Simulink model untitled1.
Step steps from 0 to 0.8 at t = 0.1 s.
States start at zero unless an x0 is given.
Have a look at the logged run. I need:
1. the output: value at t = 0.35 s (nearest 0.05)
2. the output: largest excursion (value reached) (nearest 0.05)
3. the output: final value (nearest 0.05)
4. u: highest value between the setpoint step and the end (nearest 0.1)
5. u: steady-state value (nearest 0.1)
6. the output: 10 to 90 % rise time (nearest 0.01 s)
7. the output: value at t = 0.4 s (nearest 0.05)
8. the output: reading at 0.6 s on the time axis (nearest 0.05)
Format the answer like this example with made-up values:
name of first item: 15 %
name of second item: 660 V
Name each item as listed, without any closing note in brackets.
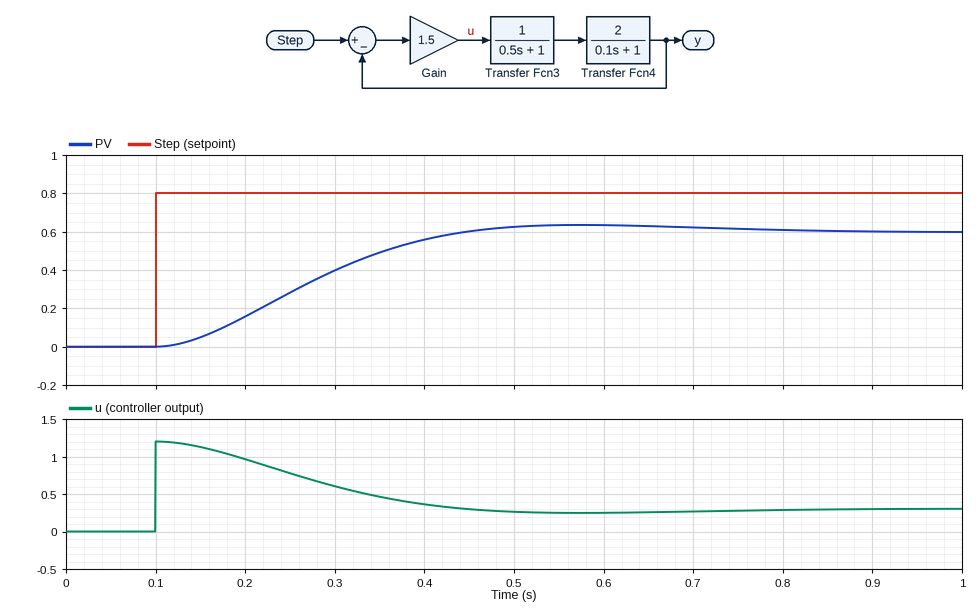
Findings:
the output: value at t = 0.35 s: 0.50
the output: largest excursion (value reached): 0.65
the output: final value: 0.60
u: highest value between the setpoint step and the end: 1.2
u: steady-state value: 0.3
the output: 10 to 90 % rise time: 0.23 s
the output: value at t = 0.4 s: 0.55
the output: reading at 0.6 s on the time axis: 0.65
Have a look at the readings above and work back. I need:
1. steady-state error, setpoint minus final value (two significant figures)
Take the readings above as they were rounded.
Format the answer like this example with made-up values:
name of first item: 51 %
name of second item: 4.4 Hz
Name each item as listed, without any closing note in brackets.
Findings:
steady-state error, setpoint minus final value: 0.20
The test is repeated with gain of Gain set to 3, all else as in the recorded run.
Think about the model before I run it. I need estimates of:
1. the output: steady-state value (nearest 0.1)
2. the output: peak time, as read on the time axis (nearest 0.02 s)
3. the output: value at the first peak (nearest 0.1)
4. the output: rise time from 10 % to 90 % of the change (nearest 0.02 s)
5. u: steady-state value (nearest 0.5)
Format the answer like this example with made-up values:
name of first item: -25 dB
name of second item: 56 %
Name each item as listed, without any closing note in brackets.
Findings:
the output: steady-state value: 0.7
the output: peak time, as read on the time axis: 0.40 s
the output: value at the first peak: 0.8
the output: rise time from 10 % to 90 % of the change: 0.14 s
u: steady-state value: 0.5
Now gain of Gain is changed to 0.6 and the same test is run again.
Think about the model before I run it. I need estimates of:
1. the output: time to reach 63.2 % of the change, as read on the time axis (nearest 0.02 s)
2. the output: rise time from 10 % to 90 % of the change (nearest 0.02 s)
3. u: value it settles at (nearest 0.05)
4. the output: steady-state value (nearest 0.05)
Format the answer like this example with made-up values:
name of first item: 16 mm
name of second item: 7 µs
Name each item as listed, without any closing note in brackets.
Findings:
the output: time to reach 63.2 % of the change, as read on the time axis: 0.40 s
the output: rise time from 10 % to 90 % of the change: 0.44 s
u: value it settles at: 0.20
the output: steady-state value: 0.45
